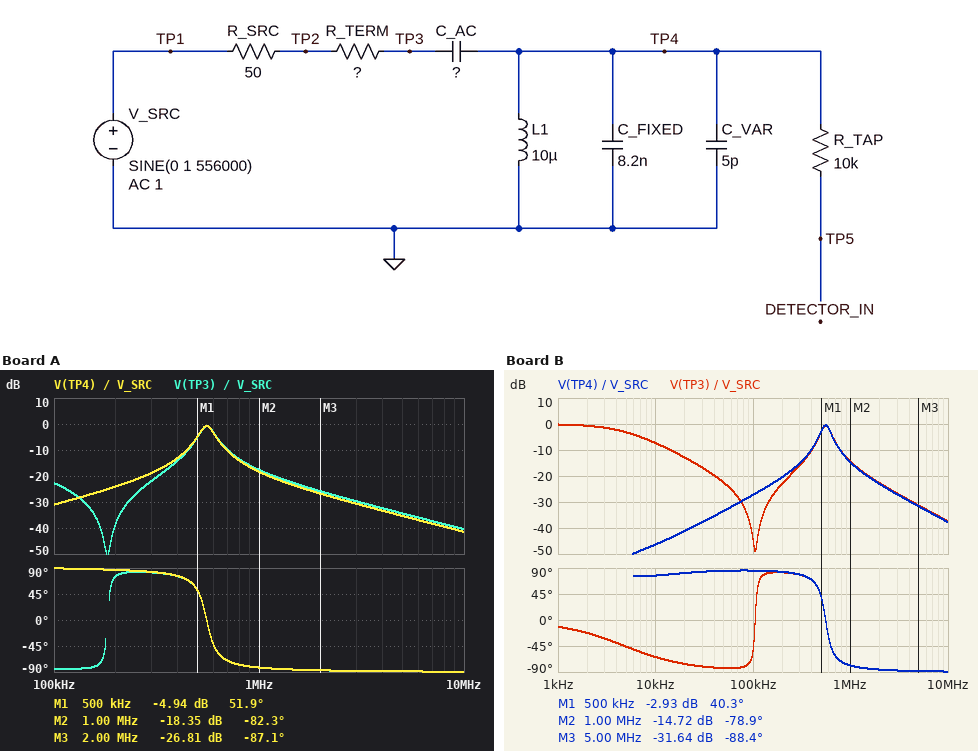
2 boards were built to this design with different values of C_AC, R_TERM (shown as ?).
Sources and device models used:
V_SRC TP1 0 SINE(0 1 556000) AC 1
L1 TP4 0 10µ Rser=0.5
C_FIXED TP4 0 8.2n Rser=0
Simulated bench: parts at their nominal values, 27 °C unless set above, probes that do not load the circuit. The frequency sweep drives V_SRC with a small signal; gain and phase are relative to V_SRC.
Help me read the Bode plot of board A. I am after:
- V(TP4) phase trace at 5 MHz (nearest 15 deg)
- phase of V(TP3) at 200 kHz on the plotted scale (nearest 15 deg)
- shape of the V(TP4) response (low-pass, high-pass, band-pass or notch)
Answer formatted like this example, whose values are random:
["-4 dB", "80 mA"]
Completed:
["-90 deg", "75 deg", "band-pass"]
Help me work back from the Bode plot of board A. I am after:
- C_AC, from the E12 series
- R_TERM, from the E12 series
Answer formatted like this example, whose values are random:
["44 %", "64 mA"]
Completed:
["68 nF", "180 Ω"]
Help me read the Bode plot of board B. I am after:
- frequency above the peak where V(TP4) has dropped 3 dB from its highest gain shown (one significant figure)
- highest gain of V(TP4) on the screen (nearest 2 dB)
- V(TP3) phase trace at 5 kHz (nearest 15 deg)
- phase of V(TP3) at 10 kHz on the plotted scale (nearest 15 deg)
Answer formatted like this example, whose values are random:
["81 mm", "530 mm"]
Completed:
["600 kHz", "0 dB", "-45 deg", "-60 deg"]
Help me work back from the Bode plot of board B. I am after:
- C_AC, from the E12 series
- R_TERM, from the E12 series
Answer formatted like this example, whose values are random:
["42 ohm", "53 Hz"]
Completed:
["220 nF", "100 Ω"]
